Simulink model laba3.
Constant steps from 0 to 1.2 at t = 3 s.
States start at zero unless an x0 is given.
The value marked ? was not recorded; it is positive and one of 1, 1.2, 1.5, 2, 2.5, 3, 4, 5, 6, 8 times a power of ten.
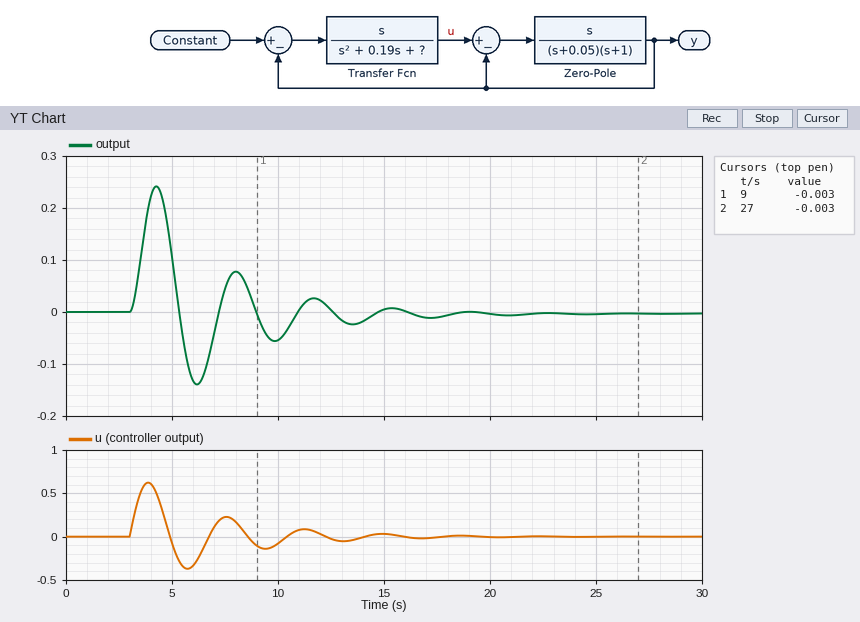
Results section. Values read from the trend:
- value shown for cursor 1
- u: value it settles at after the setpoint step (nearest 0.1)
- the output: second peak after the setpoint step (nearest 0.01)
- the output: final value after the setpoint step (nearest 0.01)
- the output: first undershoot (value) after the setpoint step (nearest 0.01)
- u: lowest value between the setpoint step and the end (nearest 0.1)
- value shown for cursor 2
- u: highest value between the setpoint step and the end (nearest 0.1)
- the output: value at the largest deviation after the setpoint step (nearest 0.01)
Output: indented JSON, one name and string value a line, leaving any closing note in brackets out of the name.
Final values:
{
  "value shown for cursor 1": "-0.003",
  "u: value it settles at after the setpoint step": "0.0",
  "the output: second peak after the setpoint step": "0.08",
  "the output: final value after the setpoint step": "0.00",
  "the output: first undershoot (value) after the setpoint step": "-0.14",
  "u: lowest value between the setpoint step and the end": "-0.4",
  "value shown for cursor 2": "-0.003",
  "u: highest value between the setpoint step and the end": "0.6",
  "the output: value at the largest deviation after the setpoint step": "0.24"
}
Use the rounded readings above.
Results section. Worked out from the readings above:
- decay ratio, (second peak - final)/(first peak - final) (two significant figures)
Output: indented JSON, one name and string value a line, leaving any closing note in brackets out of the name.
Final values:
{
  "decay ratio, (second peak - final)/(first peak - final)": "0.33"
}
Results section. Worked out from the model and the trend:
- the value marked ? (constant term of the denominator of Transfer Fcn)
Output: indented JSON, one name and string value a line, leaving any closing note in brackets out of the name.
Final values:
{
  "the value marked ?": "2.5"
}
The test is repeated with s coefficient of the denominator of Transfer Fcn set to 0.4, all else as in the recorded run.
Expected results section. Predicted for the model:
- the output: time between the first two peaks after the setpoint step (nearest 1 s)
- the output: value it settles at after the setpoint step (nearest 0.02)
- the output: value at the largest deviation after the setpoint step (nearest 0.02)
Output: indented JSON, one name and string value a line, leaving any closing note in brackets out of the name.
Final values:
{
  "the output: time between the first two peaks after the setpoint step": "4 s",
  "the output: value it settles at after the setpoint step": "0.00",
  "the output: value at the largest deviation after the setpoint step": "0.22"
}
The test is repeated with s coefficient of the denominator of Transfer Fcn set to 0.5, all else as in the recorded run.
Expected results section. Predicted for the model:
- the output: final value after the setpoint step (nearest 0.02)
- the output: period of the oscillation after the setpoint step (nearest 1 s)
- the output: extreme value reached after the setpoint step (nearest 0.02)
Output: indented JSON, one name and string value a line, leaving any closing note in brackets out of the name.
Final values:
{
  "the output: final value after the setpoint step": "0.00",
  "the output: period of the oscillation after the setpoint step": "4 s",
  "the output: extreme value reached after the setpoint step": "0.22"
}
